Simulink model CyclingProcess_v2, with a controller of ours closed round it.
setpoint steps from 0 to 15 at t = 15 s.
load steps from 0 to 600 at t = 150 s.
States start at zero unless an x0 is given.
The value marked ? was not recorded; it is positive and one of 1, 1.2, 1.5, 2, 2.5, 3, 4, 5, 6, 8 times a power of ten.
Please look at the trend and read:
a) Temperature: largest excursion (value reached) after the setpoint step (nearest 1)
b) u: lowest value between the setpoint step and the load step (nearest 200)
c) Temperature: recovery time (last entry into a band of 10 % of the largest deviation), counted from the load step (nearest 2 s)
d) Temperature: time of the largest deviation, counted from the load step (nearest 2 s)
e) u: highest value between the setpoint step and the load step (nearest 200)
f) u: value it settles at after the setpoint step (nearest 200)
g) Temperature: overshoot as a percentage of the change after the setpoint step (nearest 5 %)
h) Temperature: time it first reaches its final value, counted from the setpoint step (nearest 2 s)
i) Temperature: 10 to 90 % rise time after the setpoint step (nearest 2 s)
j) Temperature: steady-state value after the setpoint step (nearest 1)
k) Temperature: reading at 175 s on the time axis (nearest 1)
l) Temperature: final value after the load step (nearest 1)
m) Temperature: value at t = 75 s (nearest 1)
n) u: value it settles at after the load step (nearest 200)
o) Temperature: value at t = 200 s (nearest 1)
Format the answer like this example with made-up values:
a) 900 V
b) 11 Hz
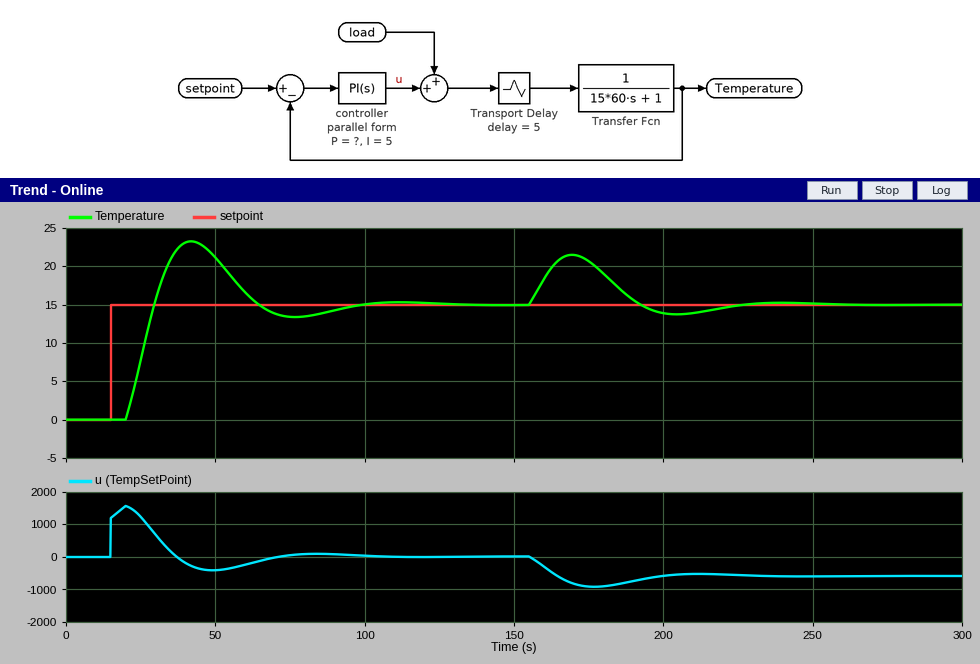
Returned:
a) 23
b) -400
c) 66 s
d) 20 s
e) 1600
f) 0
g) 55 %
h) 14 s
i) 8 s
j) 15
k) 21
l) 15
m) 13
n) -600
o) 14
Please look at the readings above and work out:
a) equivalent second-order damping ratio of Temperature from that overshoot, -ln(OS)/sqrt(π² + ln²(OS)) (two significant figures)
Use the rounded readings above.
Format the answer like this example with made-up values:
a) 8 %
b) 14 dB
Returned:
a) 0.19
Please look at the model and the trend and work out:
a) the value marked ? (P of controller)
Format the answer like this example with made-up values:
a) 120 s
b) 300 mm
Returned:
a) 80
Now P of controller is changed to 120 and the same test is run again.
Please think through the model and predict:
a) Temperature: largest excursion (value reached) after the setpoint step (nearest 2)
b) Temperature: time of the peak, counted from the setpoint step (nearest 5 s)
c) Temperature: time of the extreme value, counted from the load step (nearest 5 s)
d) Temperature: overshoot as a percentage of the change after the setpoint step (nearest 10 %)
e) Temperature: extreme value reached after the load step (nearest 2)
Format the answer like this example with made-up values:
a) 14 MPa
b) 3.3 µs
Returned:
a) 22
b) 20 s
c) 15 s
d) 50 %
e) 20
